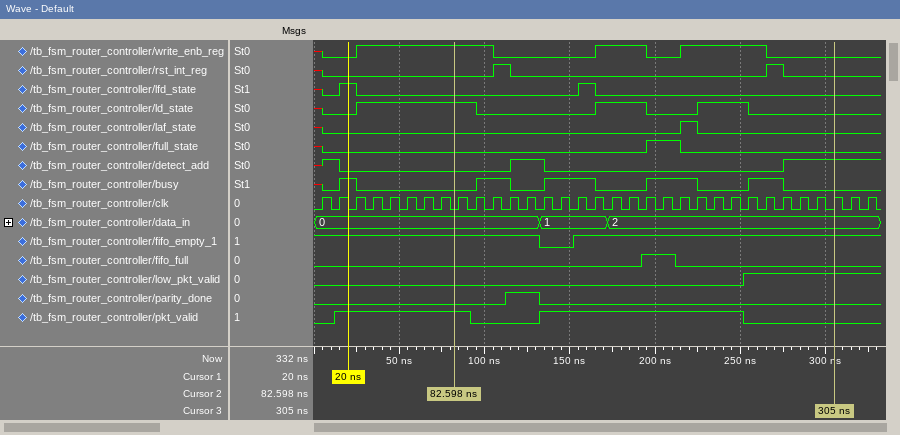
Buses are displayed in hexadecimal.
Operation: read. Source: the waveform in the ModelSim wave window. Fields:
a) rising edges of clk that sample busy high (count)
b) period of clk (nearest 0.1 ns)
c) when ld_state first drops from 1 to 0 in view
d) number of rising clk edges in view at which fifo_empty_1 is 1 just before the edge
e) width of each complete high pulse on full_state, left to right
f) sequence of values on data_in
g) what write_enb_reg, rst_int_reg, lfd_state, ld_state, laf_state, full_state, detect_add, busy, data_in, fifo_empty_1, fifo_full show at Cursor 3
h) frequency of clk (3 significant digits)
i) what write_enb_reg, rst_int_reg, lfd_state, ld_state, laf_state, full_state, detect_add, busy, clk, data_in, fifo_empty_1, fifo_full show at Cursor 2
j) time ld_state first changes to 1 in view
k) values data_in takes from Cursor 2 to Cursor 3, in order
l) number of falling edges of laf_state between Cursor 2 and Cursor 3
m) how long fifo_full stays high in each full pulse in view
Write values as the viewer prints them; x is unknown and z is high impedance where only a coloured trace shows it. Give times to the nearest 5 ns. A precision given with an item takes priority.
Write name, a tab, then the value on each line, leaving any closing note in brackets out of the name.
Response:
rising edges of clk that sample busy high	11
period of clk	10 ns
when ld_state first drops from 1 to 0 in view	95 ns
number of rising clk edges in view at which fifo_empty_1 is 1 just before the edge	31
width of each complete high pulse on full_state, left to right	20 ns
sequence of values on data_in	0, 1, 2
what write_enb_reg, rst_int_reg, lfd_state, ld_state, laf_state, full_state, detect_add, busy, data_in, fifo_empty_1, fifo_full show at Cursor 3	write_enb_reg=0, rst_int_reg=0, lfd_state=0, ld_state=0, laf_state=0, full_state=0, detect_add=1, busy=0, data_in=2, fifo_empty_1=1, fifo_full=0
frequency of clk	100 MHz
what write_enb_reg, rst_int_reg, lfd_state, ld_state, laf_state, full_state, detect_add, busy, clk, data_in, fifo_empty_1, fifo_full show at Cursor 2	write_enb_reg=1, rst_int_reg=0, lfd_state=0, ld_state=1, laf_state=0, full_state=0, detect_add=0, busy=0, clk=0, data_in=0, fifo_empty_1=1, fifo_full=0
time ld_state first changes to 1 in view	25 ns
values data_in takes from Cursor 2 to Cursor 3, in order	0, 1, 2
number of falling edges of laf_state between Cursor 2 and Cursor 3	1
how long fifo_full stays high in each full pulse in view	20 ns
